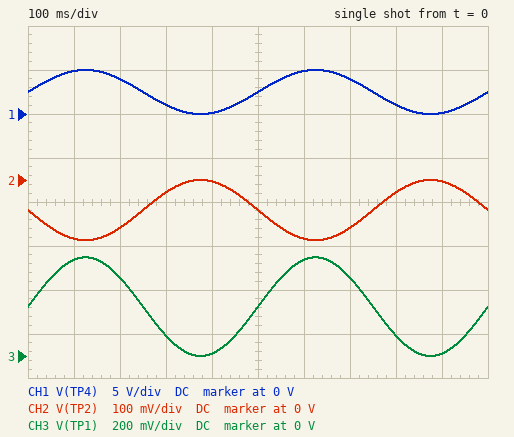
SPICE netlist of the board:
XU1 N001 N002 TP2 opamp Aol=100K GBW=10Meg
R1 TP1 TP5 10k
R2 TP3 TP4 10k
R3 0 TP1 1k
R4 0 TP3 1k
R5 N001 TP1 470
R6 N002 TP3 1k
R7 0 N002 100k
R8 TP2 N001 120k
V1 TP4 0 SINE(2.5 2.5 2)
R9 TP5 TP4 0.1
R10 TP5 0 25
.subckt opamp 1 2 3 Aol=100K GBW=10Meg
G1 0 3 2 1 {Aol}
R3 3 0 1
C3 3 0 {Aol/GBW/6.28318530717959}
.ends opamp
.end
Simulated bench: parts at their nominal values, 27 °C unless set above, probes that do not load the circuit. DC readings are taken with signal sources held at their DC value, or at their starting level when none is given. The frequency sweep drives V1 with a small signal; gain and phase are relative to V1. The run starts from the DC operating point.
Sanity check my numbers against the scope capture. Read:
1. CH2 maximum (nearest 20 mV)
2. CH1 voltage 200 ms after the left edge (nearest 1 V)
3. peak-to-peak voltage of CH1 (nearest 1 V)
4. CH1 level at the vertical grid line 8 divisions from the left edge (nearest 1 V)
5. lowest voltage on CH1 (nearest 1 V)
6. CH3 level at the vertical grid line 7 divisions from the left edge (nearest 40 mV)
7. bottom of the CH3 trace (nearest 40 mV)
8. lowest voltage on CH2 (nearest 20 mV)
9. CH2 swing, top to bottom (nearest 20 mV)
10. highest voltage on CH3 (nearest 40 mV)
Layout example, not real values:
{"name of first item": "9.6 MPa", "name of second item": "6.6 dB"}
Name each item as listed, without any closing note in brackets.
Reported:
{"CH2 maximum": "0 V", "CH1 voltage 200 ms after the left edge": "4 V", "peak-to-peak voltage of CH1": "5 V", "CH1 level at the vertical grid line 8 divisions from the left edge": "1 V", "lowest voltage on CH1": "0 V", "CH3 level at the vertical grid line 7 divisions from the left edge": "360 mV", "bottom of the CH3 trace": "0 V", "lowest voltage on CH2": "-140 mV", "CH2 swing, top to bottom": "140 mV", "highest voltage on CH3": "440 mV"}
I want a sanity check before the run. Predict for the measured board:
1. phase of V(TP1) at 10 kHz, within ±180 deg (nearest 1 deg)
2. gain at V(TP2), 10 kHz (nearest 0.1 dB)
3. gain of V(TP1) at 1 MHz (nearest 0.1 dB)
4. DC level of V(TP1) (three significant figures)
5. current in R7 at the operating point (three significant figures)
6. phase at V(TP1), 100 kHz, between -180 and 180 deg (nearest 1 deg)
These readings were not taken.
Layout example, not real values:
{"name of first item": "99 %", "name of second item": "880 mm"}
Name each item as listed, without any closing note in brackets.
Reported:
{"phase of V(TP1) at 10 kHz, within ±180 deg": "0 deg", "gain at V(TP2), 10 kHz": "-31.3 dB", "gain of V(TP1) at 1 MHz": "-20.9 dB", "DC level of V(TP1)": "224 mV", "current in R7 at the operating point": "2.23 µA", "phase at V(TP1), 100 kHz, between -180 and 180 deg": "0 deg"}
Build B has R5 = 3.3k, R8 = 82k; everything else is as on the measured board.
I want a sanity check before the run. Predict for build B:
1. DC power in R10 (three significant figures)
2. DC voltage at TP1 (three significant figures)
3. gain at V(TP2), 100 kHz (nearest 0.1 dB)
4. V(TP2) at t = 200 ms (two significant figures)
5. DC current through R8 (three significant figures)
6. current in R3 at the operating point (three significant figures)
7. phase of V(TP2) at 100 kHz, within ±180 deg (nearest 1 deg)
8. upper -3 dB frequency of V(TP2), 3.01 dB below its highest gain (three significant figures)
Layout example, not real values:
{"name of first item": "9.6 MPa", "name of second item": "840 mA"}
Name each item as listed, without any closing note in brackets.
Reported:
{"DC power in R10": "248 mW", "DC voltage at TP1": "226 mV", "gain at V(TP2), 100 kHz": "-24.2 dB", "V(TP2) at t = 200 ms": "250 mV", "DC current through R8": "796 nA", "current in R3 at the operating point": "226 µA", "phase of V(TP2) at 100 kHz, within ±180 deg": "-12 deg", "upper -3 dB frequency of V(TP2), 3.01 dB below its highest gain": "488 kHz"}
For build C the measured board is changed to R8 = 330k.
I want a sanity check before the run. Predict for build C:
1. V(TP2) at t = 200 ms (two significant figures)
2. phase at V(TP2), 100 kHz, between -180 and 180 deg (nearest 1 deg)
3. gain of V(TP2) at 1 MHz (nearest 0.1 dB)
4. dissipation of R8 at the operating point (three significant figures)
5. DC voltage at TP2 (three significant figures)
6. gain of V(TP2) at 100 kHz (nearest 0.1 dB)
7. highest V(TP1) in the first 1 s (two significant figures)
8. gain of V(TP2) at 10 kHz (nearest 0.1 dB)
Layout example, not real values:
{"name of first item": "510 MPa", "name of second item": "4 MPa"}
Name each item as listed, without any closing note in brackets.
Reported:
{"V(TP2) at t = 200 ms": "-920 mV", "phase at V(TP2), 100 kHz, between -180 and 180 deg": "113 deg", "gain of V(TP2) at 1 MHz": "-40.3 dB", "dissipation of R8 at the operating point": "1.94 µW", "DC voltage at TP2": "-577 mV", "gain of V(TP2) at 100 kHz": "-21.0 dB", "highest V(TP1) in the first 1 s": "450 mV", "gain of V(TP2) at 10 kHz": "-13.0 dB"}
